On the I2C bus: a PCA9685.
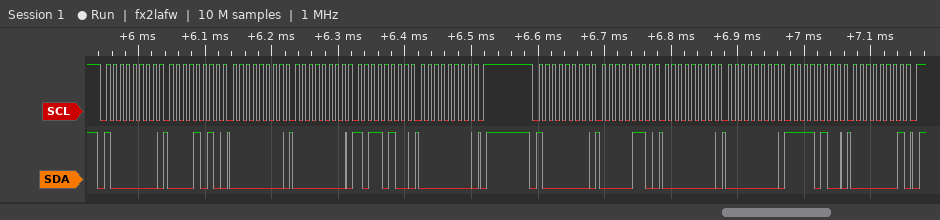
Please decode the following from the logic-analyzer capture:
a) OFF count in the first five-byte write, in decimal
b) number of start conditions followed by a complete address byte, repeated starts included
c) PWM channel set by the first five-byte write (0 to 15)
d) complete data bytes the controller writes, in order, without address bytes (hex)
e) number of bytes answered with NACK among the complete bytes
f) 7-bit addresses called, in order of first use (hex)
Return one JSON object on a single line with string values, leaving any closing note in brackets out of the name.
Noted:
{"OFF count in the first five-byte write, in decimal": "180", "number of start conditions followed by a complete address byte, repeated starts included": "2", "PWM channel set by the first five-byte write": "1", "complete data bytes the controller writes, in order, without address bytes": "0A 00 00 B4 00 06 00 00 F4 01", "number of bytes answered with NACK among the complete bytes": "0", "7-bit addresses called, in order of first use": "0x40"}
